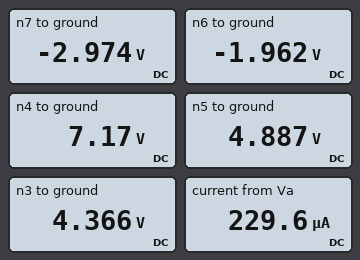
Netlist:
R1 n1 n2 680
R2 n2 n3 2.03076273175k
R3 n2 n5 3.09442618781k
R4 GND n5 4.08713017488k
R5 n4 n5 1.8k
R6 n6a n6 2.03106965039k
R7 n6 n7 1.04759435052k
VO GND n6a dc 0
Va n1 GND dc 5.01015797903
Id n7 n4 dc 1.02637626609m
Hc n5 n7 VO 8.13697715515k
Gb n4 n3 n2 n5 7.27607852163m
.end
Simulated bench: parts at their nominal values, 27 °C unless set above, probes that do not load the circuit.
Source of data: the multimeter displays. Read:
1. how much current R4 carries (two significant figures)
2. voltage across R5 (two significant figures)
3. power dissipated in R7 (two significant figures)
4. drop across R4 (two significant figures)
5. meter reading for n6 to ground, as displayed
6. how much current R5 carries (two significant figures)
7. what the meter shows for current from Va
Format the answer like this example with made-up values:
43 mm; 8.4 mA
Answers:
1.2 mA; 2.3 V; 980 µW; 4.9 V; -1.962 V; 1.3 mA; 229.6 µA
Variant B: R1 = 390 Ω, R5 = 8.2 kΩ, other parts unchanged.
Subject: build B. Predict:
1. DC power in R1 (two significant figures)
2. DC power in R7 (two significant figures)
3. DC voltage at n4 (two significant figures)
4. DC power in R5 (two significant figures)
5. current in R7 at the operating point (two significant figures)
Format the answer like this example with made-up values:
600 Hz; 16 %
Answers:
21 µW; 1.0 mW; 15 V; 13 mW; 980 µA
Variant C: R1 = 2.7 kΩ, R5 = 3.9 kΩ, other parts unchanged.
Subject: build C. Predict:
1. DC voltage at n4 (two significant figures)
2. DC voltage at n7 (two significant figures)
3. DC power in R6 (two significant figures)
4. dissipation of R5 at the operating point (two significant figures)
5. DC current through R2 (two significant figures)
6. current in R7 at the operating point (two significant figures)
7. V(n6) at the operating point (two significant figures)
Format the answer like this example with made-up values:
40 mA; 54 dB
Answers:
9.3 V; -2.7 V; 1.6 mW; 6.1 mW; 220 µA; 880 µA; -1.8 V
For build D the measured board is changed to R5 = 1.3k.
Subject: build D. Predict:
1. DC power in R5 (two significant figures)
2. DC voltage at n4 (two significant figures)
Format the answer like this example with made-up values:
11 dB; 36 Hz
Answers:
2.1 mW; 6.5 V
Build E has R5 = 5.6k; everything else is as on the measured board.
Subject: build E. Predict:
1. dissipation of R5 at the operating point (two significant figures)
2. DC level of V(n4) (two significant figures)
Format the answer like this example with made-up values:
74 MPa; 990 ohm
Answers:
9.0 mW; 12 V
